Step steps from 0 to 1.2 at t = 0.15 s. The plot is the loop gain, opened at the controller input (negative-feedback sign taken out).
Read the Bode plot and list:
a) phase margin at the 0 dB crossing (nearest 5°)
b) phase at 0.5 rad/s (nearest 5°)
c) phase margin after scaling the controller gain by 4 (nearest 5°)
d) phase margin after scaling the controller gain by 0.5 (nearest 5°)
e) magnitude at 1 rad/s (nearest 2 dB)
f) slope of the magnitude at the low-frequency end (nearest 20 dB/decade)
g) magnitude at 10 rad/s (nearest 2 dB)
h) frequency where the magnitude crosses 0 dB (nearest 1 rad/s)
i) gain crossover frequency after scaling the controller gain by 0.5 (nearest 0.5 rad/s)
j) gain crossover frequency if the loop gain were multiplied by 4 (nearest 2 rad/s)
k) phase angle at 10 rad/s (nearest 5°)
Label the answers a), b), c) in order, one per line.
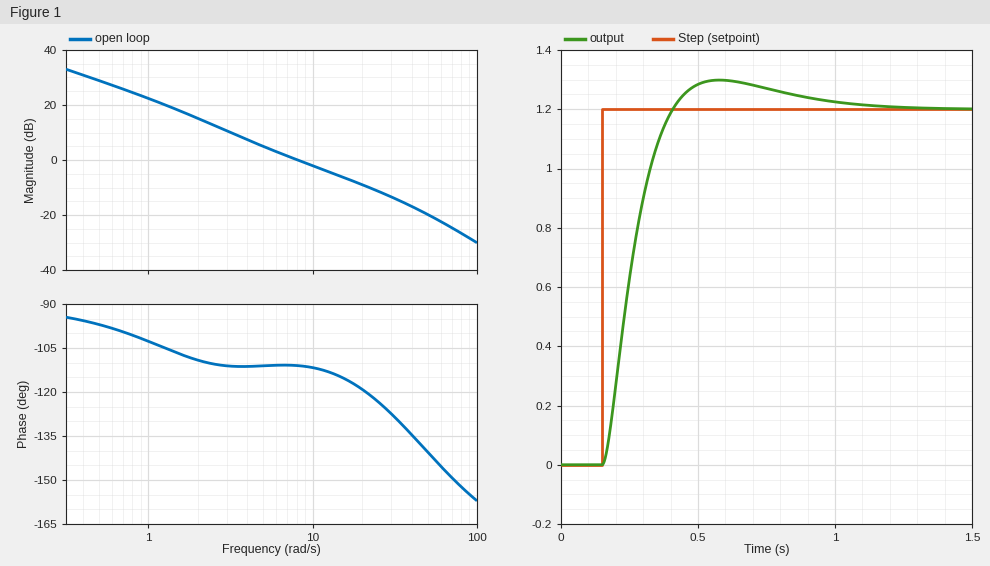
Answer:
a) 70°
b) -95°
c) 55°
d) 70°
e) 22 dB
f) -20 dB/decade
g) -2 dB
h) 8 rad/s
i) 4.5 rad/s
j) 26 rad/s
k) -110°
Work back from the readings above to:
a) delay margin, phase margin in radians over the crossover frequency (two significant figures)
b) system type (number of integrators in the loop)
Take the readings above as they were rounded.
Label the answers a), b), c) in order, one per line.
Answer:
a) 0.15 s
b) 1
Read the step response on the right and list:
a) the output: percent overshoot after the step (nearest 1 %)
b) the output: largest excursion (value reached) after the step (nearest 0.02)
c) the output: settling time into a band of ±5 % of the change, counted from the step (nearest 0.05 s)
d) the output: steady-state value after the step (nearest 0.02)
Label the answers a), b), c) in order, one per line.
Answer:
a) 8 %
b) 1.30
c) 0.65 s
d) 1.20
